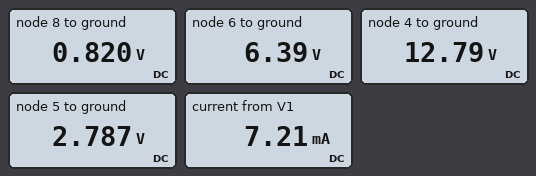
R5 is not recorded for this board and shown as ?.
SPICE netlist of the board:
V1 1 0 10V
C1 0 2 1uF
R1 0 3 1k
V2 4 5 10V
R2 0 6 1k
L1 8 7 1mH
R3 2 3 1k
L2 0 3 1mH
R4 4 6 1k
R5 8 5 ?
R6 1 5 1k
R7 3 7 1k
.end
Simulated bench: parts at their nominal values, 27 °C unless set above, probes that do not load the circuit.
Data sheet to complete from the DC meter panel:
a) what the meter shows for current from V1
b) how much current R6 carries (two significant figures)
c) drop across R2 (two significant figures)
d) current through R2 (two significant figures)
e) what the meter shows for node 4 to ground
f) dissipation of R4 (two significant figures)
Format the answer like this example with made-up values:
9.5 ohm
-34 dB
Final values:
7.21 mA
7.2 mA
6.4 V
6.4 mA
12.79 V
41 mW
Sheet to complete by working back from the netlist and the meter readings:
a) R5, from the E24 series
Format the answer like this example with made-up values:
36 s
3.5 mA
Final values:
2.4 kΩ
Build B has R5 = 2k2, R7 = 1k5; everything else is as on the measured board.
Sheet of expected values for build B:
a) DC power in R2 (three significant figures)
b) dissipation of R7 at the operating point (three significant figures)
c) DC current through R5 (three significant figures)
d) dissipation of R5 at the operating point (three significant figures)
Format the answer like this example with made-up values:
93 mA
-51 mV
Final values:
41.1 mW
874 µW
763 µA
1.28 mW
